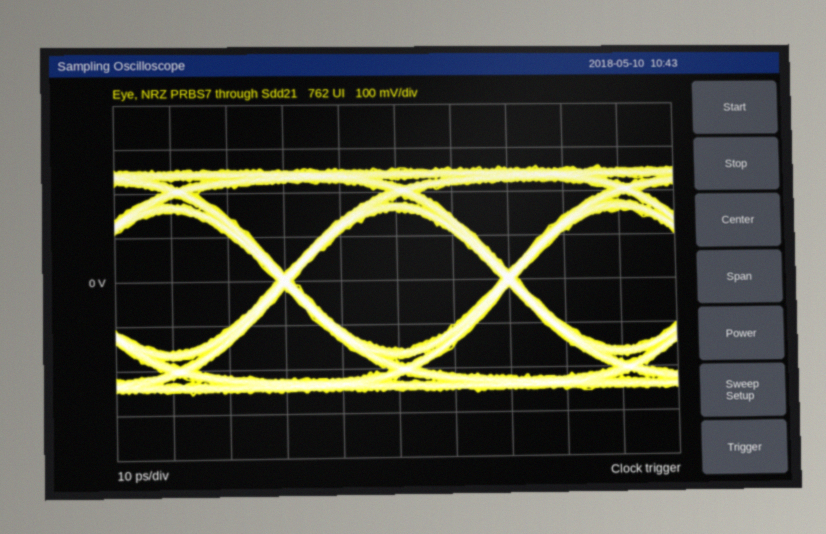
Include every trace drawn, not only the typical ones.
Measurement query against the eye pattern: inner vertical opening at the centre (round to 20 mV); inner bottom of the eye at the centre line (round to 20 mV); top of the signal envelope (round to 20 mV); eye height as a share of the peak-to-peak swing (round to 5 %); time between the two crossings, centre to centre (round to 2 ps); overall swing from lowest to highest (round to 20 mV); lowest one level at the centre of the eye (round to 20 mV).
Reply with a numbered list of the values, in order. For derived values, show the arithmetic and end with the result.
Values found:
1. 320 mV
2. -160 mV
3. 260 mV
4. 320 mV / 520 mV ≈ 61.5 %, so 60 % to the nearest 5 %
5. 40 ps
6. 520 mV
7. 160 mV
